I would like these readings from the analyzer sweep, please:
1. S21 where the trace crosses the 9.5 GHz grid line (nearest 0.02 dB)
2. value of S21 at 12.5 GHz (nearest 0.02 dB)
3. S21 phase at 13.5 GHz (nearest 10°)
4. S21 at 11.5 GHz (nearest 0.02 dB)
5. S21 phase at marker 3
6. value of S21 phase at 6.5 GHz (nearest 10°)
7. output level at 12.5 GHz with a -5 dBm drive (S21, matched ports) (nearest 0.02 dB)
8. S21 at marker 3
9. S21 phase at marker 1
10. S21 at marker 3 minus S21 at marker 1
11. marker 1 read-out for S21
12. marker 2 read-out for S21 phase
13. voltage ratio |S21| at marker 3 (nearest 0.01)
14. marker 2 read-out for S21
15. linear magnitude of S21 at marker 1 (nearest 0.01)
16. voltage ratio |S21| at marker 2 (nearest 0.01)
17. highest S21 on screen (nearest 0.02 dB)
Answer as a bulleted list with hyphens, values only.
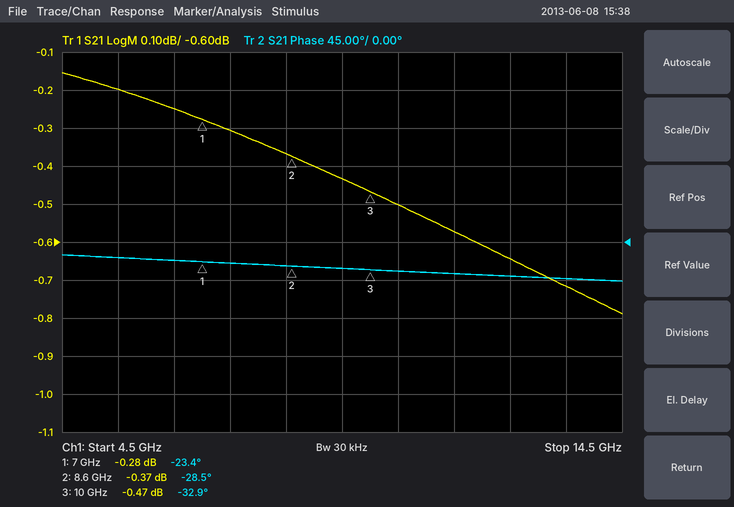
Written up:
- -0.44 dB
- -0.64 dB
- -40°
- -0.58 dB
- -32.9°
- -20°
- -5.64 dBm
- -0.47 dB
- -23.4°
- -0.19 dB
- -0.28 dB
- -28.5°
- 0.95
- -0.37 dB
- 0.97
- 0.96
- -0.16 dB
